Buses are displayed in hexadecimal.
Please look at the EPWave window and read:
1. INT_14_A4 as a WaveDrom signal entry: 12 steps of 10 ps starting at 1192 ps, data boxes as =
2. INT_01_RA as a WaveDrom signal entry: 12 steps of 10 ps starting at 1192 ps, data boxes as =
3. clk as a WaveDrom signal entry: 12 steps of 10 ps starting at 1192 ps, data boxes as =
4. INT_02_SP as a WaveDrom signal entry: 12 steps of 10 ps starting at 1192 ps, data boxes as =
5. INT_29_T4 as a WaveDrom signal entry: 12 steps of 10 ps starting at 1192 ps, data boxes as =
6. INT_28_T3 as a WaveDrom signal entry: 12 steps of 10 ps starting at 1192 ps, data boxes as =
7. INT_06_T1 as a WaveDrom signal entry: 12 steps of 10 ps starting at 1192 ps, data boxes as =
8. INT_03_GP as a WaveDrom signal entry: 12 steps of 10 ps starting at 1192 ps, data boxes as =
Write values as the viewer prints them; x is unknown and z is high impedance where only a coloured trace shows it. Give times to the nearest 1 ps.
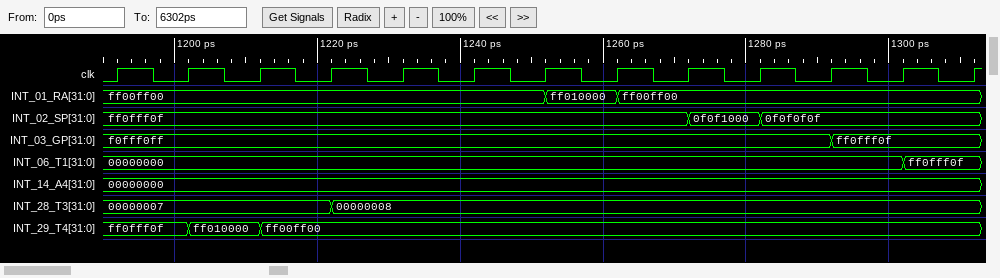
{name: 'INT_14_A4', wave: '=...........', data: '00000000'}
{name: 'INT_01_RA', wave: '=.....==....', data: 'ff00ff00 ff010000 ff00ff00'}
{name: 'clk', wave: 'p...........'}
{name: 'INT_02_SP', wave: '=.......==..', data: 'ff0fff0f 0f0f1000 0f0f0f0f'}
{name: 'INT_29_T4', wave: '===.........', data: 'ff0fff0f ff010000 ff00ff00'}
{name: 'INT_28_T3', wave: '=..=........', data: '00000007 00000008'}
{name: 'INT_06_T1', wave: '=..........=', data: '00000000 ff0fff0f'}
{name: 'INT_03_GP', wave: '=.........=.', data: 'f0fff0ff ff0fff0f'}
